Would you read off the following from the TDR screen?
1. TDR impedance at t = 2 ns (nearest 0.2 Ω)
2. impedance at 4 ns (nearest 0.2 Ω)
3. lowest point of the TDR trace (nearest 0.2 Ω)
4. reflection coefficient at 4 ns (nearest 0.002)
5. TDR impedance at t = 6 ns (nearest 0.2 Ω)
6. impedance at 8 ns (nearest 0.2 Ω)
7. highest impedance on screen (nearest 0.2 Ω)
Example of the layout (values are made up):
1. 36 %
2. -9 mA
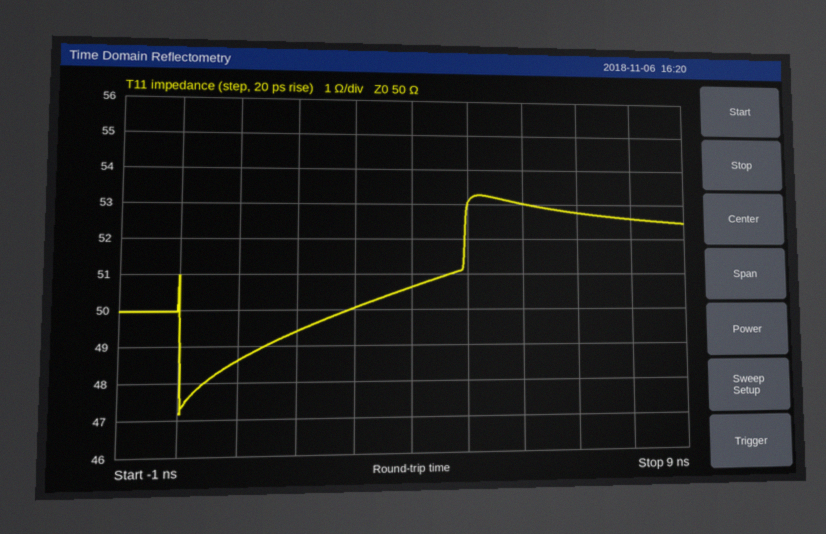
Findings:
1. 49.4 Ω
2. 50.6 Ω
3. 47.2 Ω
4. +0.006
5. 53.0 Ω
6. 52.6 Ω
7. 53.2 Ω
